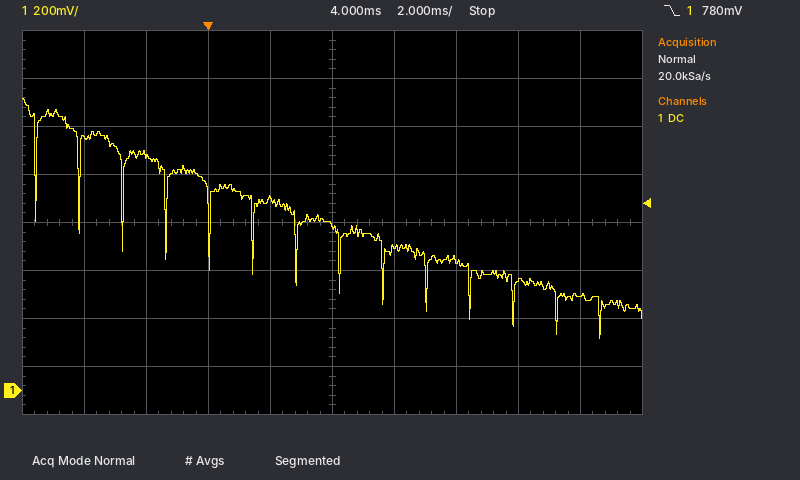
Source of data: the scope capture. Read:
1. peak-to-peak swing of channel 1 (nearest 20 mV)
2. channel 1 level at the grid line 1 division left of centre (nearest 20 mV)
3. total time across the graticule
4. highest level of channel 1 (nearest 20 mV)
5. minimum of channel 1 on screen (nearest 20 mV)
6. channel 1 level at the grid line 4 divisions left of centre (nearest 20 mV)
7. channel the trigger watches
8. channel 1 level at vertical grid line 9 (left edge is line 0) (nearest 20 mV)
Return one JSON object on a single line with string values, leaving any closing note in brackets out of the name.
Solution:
{"peak-to-peak swing of channel 1": "1.00 V", "channel 1 level at the grid line 1 division left of centre": "800 mV", "total time across the graticule": "20 ms", "highest level of channel 1": "1.22 V", "minimum of channel 1 on screen": "220 mV", "channel 1 level at the grid line 4 divisions left of centre": "1.06 V", "channel the trigger watches": "channel 1", "channel 1 level at vertical grid line 9 (left edge is line 0)": "400 mV"}
